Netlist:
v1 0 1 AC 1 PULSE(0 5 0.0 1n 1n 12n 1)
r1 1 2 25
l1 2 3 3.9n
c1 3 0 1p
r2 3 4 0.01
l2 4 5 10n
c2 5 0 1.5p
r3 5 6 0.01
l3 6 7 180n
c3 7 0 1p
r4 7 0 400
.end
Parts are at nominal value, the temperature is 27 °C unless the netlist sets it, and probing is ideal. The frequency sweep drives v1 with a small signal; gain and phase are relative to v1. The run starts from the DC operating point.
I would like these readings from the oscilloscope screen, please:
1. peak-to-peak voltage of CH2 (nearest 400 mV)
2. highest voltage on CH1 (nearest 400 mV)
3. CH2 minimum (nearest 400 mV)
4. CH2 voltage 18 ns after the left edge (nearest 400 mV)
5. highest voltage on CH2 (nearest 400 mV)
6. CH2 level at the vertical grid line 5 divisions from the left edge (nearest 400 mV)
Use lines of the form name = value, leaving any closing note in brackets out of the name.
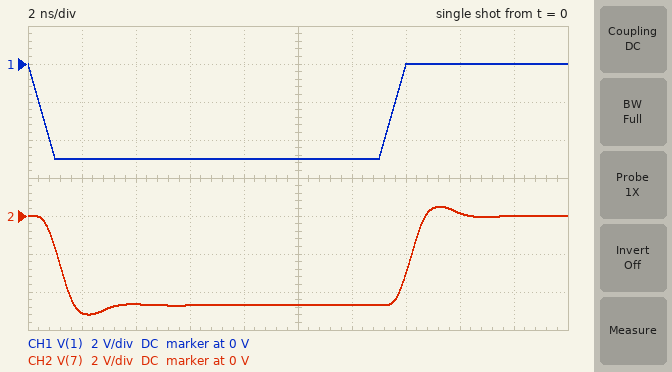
peak-to-peak voltage of CH2 = 5.6 V
highest voltage on CH1 = 0 V
CH2 minimum = -5.2 V
CH2 voltage 18 ns after the left edge = 0 V
highest voltage on CH2 = 400 mV
CH2 level at the vertical grid line 5 divisions from the left edge = -4.8 V
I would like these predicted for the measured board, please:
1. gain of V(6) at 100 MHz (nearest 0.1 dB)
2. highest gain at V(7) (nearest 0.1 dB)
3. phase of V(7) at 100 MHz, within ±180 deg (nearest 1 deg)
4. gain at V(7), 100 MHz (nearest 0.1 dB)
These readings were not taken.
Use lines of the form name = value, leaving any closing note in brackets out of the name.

gain of V(6) at 100 MHz = -0.5 dB
highest gain at V(7) = 0.5 dB
phase of V(7) at 100 MHz, within ±180 deg = 160 deg
gain at V(7), 100 MHz = -0.2 dB
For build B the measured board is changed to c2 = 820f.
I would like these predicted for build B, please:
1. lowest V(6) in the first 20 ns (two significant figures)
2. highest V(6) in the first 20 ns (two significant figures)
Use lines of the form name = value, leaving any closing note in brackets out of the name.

lowest V(6) in the first 20 ns = -5.2 V
highest V(6) in the first 20 ns = 480 mV
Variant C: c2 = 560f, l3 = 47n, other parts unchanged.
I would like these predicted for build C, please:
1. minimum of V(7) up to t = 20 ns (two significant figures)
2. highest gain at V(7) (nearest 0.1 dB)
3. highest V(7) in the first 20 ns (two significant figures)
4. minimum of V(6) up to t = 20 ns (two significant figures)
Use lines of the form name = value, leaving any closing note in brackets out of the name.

minimum of V(7) up to t = 20 ns = -5.5 V
highest gain at V(7) = 4.0 dB
highest V(7) in the first 20 ns = 820 mV
minimum of V(6) up to t = 20 ns = -5.0 V
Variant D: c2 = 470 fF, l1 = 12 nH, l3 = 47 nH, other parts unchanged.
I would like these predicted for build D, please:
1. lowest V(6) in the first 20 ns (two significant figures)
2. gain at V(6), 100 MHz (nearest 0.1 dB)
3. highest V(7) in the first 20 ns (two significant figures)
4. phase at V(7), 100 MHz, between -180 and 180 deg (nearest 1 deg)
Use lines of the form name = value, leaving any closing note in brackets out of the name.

lowest V(6) in the first 20 ns = -5.2 V
gain at V(6), 100 MHz = -0.4 dB
highest V(7) in the first 20 ns = 1.0 V
phase at V(7), 100 MHz, between -180 and 180 deg = 172 deg
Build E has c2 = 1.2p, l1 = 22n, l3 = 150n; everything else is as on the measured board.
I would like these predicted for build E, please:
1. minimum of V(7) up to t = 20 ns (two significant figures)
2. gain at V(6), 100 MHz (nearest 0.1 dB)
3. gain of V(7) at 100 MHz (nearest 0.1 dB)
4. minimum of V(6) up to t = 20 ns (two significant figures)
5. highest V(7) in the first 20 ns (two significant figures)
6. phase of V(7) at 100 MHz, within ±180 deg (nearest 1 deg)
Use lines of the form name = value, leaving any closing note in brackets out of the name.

minimum of V(7) up to t = 20 ns = -5.5 V
gain at V(6), 100 MHz = -0.4 dB
gain of V(7) at 100 MHz = -0.1 dB
minimum of V(6) up to t = 20 ns = -5.3 V
highest V(7) in the first 20 ns = 790 mV
phase of V(7) at 100 MHz, within ±180 deg = 161 deg
